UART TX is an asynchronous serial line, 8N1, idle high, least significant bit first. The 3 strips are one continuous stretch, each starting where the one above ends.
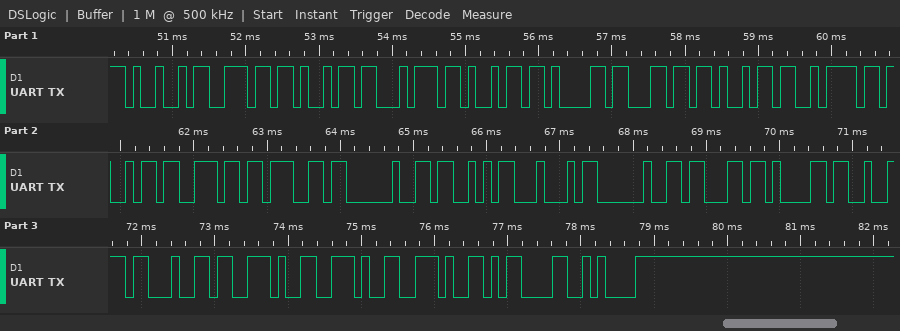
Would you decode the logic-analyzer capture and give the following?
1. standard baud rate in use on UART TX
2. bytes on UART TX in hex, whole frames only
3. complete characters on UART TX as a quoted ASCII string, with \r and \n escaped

9600 baud
49 6E 69 74 69 61 6C 69 7A 69 6E 67 20 53 44 20 63 61 72 64 2E 2E 2E 0D 0A
"Initializing SD card...\r\n"
